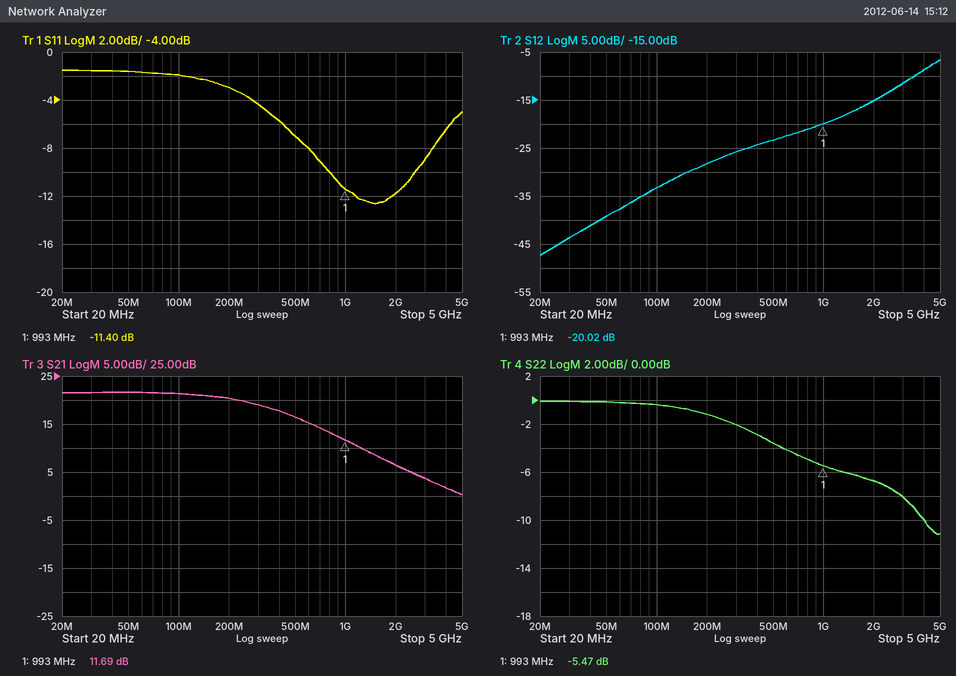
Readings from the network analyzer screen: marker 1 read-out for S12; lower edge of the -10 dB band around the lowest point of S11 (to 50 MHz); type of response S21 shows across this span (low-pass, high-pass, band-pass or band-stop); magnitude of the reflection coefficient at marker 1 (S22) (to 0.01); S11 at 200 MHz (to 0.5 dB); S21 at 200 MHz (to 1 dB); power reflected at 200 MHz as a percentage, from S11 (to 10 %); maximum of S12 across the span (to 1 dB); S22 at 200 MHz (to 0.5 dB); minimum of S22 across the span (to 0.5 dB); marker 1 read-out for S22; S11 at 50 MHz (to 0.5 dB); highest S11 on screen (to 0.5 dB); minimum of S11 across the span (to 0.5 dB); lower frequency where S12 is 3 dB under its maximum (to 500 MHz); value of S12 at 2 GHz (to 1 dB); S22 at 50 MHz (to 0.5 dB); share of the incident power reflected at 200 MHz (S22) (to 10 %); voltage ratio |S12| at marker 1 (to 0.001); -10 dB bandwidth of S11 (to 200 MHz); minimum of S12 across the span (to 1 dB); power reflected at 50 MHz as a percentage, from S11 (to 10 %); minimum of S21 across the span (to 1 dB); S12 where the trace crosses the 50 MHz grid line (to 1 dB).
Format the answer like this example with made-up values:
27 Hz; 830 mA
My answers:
-20.02 dB; 800 MHz; low-pass; 0.53; -3.0 dB; 20 dB; 50 %; -7 dB; -1.0 dB; -11.0 dB; -5.47 dB; -1.5 dB; -1.5 dB; -12.5 dB; 3.5 GHz; -15 dB; 0.0 dB; 80 %; 0.100; 1.8 GHz; -47 dB; 70 %; 0 dB; -39 dB
